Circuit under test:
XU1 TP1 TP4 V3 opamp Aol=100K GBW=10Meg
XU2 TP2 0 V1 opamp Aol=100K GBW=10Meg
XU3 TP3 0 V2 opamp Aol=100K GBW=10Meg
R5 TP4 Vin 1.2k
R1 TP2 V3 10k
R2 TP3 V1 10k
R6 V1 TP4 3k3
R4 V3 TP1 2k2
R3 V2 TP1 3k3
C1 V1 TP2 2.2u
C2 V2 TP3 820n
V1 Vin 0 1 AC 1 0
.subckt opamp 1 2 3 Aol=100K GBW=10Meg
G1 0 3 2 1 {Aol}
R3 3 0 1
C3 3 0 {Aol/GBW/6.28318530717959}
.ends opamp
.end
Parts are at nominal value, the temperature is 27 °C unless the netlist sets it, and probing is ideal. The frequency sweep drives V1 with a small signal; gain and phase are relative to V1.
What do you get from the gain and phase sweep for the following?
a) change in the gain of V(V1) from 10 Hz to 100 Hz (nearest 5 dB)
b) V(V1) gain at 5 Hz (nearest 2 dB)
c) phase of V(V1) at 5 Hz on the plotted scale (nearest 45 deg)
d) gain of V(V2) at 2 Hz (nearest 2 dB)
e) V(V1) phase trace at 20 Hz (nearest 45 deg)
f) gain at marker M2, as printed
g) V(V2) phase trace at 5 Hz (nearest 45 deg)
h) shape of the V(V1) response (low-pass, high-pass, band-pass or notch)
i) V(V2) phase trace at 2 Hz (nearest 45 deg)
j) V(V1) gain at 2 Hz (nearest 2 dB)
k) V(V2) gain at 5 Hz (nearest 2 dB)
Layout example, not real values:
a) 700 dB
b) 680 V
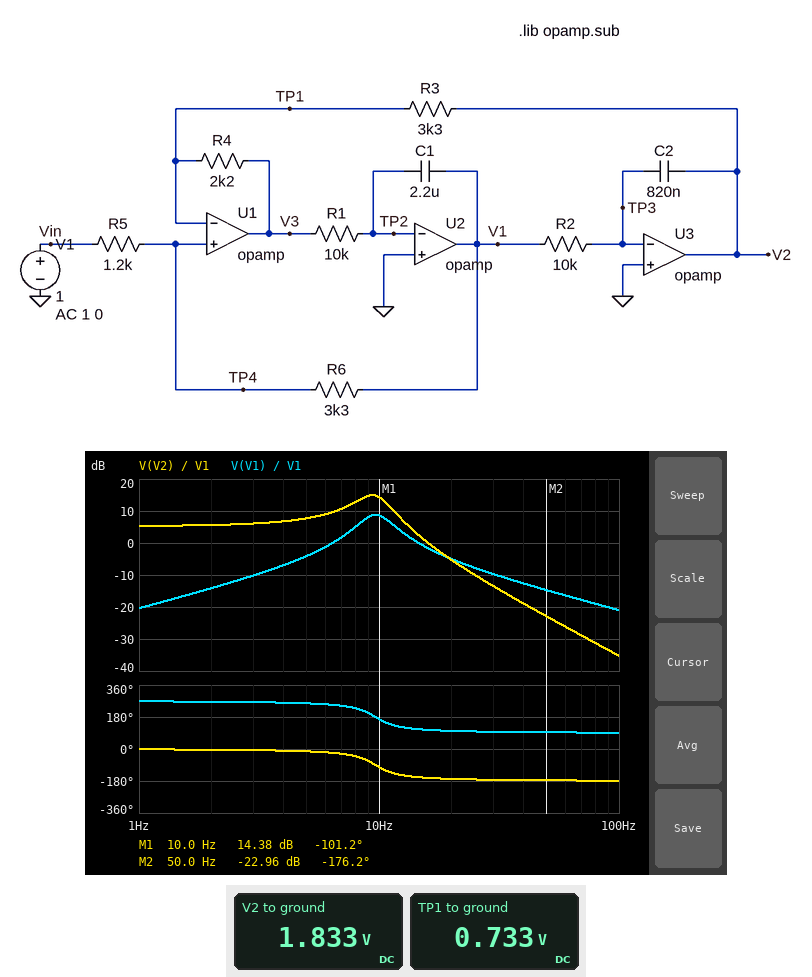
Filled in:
a) -30 dB
b) -4 dB
c) 270 deg
d) 6 dB
e) 90 deg
f) -22.96 dB
g) 0 deg
h) band-pass
i) 0 deg
j) -14 dB
k) 8 dB
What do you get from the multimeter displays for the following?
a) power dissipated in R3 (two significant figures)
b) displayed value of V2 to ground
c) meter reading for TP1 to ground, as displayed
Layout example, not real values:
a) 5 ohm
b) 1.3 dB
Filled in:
a) 370 µW
b) 1.833 V
c) 0.733 V
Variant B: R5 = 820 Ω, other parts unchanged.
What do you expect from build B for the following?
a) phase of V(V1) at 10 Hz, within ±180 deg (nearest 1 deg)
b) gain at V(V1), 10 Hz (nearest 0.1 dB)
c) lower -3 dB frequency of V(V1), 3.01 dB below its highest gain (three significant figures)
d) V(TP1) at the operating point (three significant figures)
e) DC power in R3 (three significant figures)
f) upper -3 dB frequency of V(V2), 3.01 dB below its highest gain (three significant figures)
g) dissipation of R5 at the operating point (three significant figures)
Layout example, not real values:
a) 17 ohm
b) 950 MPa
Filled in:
a) 165 deg
b) 11.8 dB
c) 8.55 Hz
d) 801 mV
e) 437 µW
f) 10.7 Hz
g) 48.3 µW
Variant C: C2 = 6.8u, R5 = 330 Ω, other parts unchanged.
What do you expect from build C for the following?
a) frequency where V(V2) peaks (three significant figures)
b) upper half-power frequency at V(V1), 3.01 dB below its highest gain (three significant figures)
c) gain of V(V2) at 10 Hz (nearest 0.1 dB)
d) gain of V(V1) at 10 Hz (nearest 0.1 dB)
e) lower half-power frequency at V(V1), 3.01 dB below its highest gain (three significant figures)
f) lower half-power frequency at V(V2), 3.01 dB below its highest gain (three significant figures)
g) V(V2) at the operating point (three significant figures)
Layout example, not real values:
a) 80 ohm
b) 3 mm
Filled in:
a) 3.27 Hz
b) 3.95 Hz
c) -10.8 dB
d) 1.8 dB
e) 2.86 Hz
f) 2.66 Hz
g) 2.27 V
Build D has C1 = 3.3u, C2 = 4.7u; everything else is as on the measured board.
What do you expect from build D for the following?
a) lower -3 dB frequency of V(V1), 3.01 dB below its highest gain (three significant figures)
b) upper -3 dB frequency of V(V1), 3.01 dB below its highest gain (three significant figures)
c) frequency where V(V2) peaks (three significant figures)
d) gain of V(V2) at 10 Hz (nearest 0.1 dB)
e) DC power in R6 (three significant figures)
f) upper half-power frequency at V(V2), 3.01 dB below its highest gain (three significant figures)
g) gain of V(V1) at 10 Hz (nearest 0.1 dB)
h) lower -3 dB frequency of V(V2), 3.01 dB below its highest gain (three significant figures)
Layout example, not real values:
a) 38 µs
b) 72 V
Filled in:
a) 2.40 Hz
b) 4.54 Hz
c) 2.93 Hz
d) -13.2 dB
e) 163 µW
f) 3.91 Hz
g) -3.8 dB
h) 1.38 Hz
